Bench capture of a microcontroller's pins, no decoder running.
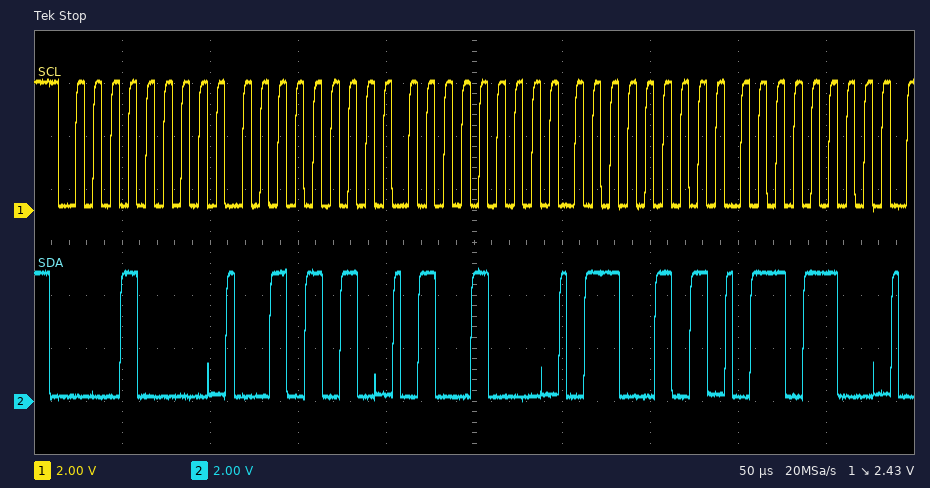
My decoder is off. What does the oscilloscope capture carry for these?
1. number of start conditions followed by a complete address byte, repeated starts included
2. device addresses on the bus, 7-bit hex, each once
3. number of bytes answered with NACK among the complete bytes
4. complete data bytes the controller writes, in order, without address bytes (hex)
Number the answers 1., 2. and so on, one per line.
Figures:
1. 1
2. 0x08
3. 0
4. 2A 48 65 6C
